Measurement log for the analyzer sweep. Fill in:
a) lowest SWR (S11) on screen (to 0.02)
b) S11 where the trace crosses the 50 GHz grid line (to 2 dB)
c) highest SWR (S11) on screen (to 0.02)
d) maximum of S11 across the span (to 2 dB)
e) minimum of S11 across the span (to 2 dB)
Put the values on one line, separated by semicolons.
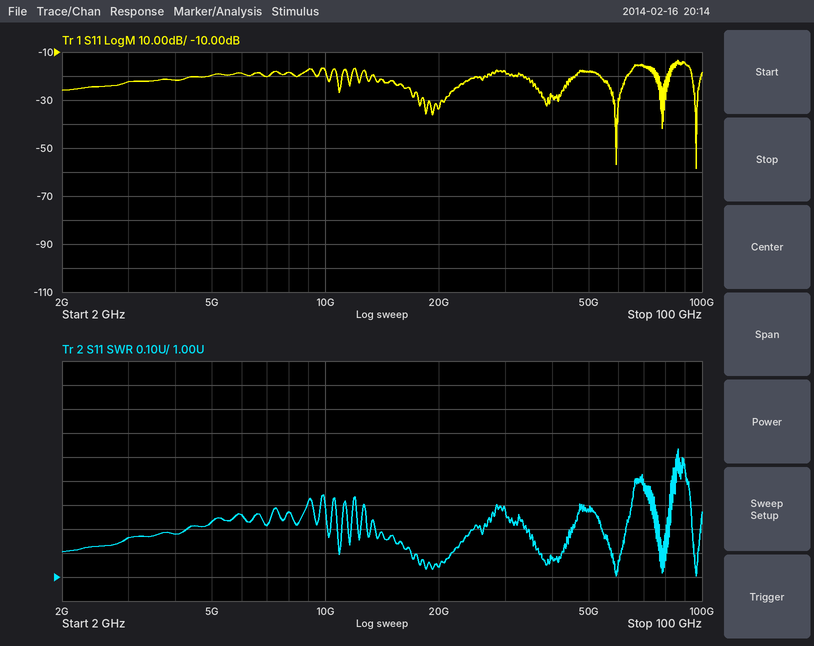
1.00; -18 dB; 1.54; -14 dB; -58 dB
